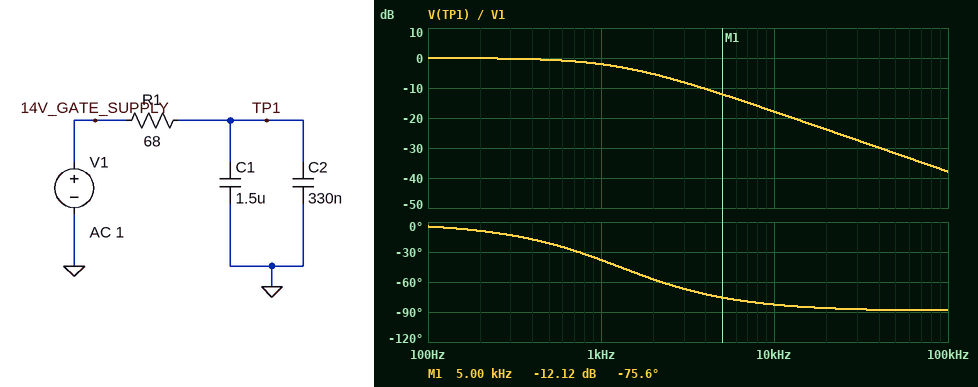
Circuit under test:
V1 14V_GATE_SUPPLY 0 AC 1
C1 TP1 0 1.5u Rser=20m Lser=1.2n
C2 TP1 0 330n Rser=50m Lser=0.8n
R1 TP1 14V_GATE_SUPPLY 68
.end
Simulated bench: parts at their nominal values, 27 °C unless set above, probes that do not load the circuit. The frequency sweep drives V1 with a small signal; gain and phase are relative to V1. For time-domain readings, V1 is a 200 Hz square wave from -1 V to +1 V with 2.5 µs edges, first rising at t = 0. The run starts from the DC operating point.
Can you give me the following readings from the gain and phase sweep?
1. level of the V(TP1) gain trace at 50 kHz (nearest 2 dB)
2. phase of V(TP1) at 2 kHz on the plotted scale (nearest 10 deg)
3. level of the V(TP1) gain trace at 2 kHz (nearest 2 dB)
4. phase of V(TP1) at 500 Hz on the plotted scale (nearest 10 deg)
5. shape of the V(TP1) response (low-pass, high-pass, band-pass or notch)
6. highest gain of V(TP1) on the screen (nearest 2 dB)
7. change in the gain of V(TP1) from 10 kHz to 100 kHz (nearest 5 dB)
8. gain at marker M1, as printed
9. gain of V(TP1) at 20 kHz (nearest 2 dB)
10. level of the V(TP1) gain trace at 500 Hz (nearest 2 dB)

-32 dB
-60 deg
-6 dB
-20 deg
low-pass
0 dB
-20 dB
-12.12 dB
-24 dB
0 dB
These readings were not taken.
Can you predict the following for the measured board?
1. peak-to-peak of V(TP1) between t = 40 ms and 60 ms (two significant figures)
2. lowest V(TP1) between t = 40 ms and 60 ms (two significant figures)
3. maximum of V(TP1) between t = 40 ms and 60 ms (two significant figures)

2.0 V
-1.0 V
1.0 V
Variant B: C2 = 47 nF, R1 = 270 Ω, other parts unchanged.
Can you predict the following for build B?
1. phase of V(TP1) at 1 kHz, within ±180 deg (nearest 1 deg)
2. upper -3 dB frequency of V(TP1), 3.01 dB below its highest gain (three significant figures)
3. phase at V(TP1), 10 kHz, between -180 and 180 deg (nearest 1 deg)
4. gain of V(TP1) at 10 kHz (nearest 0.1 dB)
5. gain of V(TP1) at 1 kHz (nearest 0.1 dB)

-69 deg
381 Hz
-88 deg
-28.4 dB
-9.0 dB
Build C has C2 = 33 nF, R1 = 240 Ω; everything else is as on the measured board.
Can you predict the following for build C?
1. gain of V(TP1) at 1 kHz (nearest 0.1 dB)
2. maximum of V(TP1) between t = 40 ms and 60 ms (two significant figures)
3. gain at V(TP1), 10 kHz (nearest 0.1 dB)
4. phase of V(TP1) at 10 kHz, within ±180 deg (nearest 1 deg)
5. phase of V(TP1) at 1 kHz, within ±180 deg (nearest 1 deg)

-8.0 dB
1.0 V
-27.3 dB
-87 deg
-67 deg
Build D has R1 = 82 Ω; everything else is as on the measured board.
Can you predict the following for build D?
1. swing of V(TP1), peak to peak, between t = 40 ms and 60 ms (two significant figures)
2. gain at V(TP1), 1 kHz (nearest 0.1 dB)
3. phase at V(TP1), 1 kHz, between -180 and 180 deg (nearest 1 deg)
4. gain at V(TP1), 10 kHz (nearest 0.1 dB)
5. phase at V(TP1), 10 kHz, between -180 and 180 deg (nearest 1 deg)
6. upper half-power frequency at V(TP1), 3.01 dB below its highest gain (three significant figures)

2.0 V
-2.8 dB
-43 deg
-19.5 dB
-84 deg
1.06 kHz
